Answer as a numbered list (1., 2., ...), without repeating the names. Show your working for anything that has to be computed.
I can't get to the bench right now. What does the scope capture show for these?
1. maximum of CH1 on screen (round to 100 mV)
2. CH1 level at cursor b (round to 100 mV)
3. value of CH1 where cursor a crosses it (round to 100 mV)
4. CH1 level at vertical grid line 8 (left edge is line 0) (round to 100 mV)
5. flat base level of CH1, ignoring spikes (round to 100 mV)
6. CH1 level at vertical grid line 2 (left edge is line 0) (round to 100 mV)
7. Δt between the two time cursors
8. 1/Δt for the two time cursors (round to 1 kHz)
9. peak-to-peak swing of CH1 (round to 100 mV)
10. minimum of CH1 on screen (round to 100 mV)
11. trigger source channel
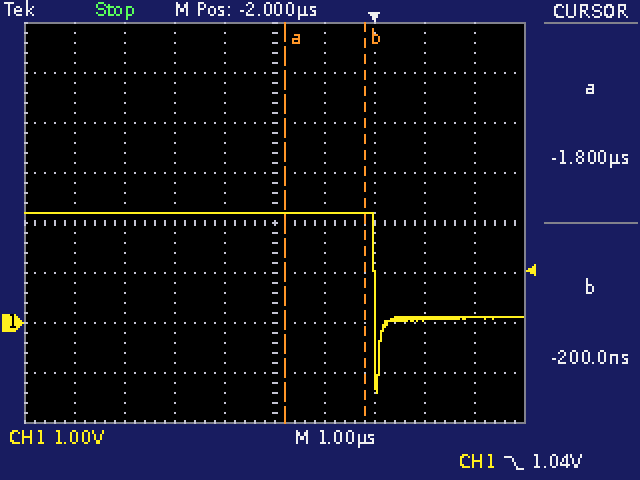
1. 2.2 V
2. 2.2 V
3. 2.2 V
4. 100 mV
5. 100 mV
6. 2.2 V
7. -200 ns − (-1.8 µs) = 1.6 µs
8. 1 / 1.6 µs ≈ 625 kHz
9. 2.2 V − (-1.4 V) = 3.6 V
10. -1.4 V
11. CH1
